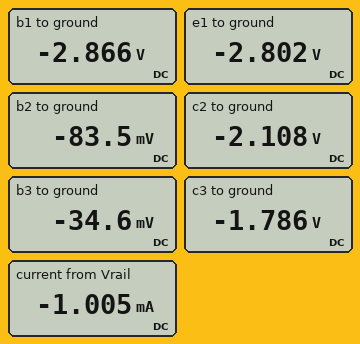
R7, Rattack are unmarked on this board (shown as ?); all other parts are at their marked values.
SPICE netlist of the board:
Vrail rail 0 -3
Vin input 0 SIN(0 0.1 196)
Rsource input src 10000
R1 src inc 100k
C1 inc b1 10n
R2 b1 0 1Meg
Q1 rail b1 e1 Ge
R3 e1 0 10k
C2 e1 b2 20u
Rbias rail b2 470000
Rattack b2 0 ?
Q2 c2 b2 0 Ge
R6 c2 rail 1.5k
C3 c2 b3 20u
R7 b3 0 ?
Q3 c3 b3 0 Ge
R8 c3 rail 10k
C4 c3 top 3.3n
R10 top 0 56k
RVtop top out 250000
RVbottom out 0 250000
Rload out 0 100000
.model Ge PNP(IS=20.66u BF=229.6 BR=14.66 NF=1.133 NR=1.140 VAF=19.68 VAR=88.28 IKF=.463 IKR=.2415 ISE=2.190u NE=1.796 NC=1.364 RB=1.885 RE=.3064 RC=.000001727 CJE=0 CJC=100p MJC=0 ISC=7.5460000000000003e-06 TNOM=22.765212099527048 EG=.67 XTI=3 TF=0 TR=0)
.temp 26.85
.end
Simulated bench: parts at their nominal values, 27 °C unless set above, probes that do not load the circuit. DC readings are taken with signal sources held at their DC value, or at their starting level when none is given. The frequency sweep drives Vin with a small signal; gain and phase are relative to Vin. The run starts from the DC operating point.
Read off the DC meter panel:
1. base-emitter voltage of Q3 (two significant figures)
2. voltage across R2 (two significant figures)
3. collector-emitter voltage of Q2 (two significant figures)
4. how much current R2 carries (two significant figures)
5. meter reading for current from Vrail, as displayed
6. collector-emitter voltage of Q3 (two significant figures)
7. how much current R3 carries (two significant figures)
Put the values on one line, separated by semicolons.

-35 mV; 2.9 V; -2.1 V; 2.9 µA; -1.005 mA; -1.8 V; 280 µA
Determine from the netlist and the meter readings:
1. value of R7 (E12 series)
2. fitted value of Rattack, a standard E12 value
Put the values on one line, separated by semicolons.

3.9 kΩ; 33 kΩ
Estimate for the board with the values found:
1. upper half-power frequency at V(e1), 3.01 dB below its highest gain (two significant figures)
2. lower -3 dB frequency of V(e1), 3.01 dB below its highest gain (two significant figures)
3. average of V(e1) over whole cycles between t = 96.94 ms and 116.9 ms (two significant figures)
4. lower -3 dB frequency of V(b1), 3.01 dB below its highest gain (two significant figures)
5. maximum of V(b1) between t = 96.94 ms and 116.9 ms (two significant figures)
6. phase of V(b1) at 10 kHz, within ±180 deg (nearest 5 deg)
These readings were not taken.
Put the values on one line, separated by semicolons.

32 kHz; 100 Hz; -2.8 V; 100 Hz; -2.8 V; -15 deg
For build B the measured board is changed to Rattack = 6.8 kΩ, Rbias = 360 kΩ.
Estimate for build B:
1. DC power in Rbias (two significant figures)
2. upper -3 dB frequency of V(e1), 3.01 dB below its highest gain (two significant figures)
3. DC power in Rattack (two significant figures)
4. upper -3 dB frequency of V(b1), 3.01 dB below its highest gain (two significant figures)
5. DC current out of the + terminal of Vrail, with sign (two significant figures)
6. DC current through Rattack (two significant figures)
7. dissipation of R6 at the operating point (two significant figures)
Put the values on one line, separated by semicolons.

24 µW; 37 kHz; 680 nW; 38 kHz; -780 µA; 10 µA; 200 µW
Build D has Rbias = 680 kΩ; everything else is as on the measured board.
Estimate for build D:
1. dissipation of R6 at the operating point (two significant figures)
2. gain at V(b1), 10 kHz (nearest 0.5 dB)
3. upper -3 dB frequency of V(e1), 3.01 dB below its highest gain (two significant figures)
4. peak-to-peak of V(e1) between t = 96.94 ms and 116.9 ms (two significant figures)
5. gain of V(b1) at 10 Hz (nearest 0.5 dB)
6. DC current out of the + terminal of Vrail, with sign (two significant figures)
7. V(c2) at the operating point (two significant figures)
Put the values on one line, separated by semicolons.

400 µW; -11.0 dB; 33 kHz; 51 mV; -30.5 dB; -930 µA; -2.2 V
